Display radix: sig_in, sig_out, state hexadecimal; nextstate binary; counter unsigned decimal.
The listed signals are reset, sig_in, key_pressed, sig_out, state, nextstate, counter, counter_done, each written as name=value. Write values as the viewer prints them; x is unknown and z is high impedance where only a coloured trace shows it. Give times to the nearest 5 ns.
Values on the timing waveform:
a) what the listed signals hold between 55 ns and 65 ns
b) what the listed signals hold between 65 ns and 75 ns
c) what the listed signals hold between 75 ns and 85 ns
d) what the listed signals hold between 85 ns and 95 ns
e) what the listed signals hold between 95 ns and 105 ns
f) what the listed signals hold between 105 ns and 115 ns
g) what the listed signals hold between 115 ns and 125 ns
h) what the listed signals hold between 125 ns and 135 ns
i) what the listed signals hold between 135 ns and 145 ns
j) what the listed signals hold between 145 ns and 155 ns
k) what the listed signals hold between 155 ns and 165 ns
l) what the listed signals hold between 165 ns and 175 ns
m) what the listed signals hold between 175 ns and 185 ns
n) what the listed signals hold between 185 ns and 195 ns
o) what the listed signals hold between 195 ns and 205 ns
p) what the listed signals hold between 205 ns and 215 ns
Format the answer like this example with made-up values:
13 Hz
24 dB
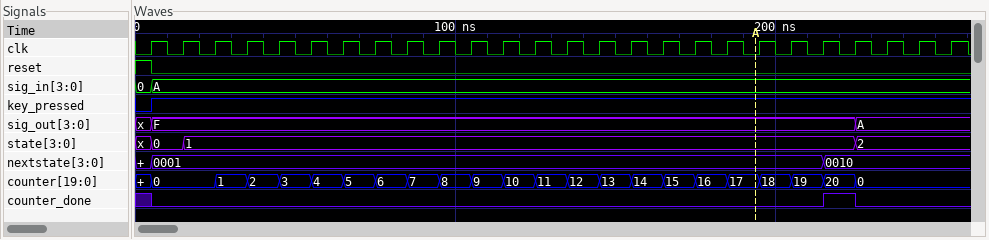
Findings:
reset=0, sig_in=A, key_pressed=1, sig_out=F, state=1, nextstate=0001, counter=4, counter_done=0
reset=0, sig_in=A, key_pressed=1, sig_out=F, state=1, nextstate=0001, counter=5, counter_done=0
reset=0, sig_in=A, key_pressed=1, sig_out=F, state=1, nextstate=0001, counter=6, counter_done=0
reset=0, sig_in=A, key_pressed=1, sig_out=F, state=1, nextstate=0001, counter=7, counter_done=0
reset=0, sig_in=A, key_pressed=1, sig_out=F, state=1, nextstate=0001, counter=8, counter_done=0
reset=0, sig_in=A, key_pressed=1, sig_out=F, state=1, nextstate=0001, counter=9, counter_done=0
reset=0, sig_in=A, key_pressed=1, sig_out=F, state=1, nextstate=0001, counter=10, counter_done=0
reset=0, sig_in=A, key_pressed=1, sig_out=F, state=1, nextstate=0001, counter=11, counter_done=0
reset=0, sig_in=A, key_pressed=1, sig_out=F, state=1, nextstate=0001, counter=12, counter_done=0
reset=0, sig_in=A, key_pressed=1, sig_out=F, state=1, nextstate=0001, counter=13, counter_done=0
reset=0, sig_in=A, key_pressed=1, sig_out=F, state=1, nextstate=0001, counter=14, counter_done=0
reset=0, sig_in=A, key_pressed=1, sig_out=F, state=1, nextstate=0001, counter=15, counter_done=0
reset=0, sig_in=A, key_pressed=1, sig_out=F, state=1, nextstate=0001, counter=16, counter_done=0
reset=0, sig_in=A, key_pressed=1, sig_out=F, state=1, nextstate=0001, counter=17, counter_done=0
reset=0, sig_in=A, key_pressed=1, sig_out=F, state=1, nextstate=0001, counter=18, counter_done=0
reset=0, sig_in=A, key_pressed=1, sig_out=F, state=1, nextstate=0001, counter=19, counter_done=0
